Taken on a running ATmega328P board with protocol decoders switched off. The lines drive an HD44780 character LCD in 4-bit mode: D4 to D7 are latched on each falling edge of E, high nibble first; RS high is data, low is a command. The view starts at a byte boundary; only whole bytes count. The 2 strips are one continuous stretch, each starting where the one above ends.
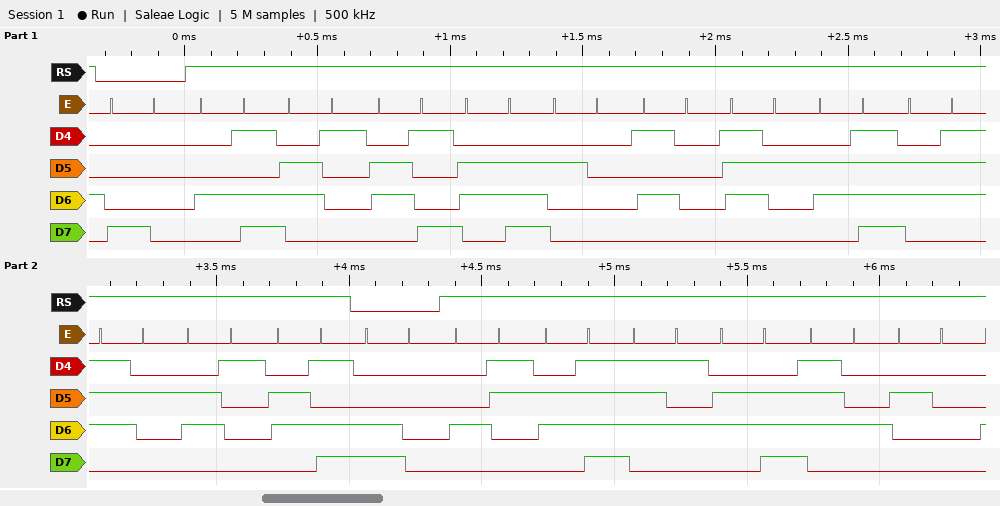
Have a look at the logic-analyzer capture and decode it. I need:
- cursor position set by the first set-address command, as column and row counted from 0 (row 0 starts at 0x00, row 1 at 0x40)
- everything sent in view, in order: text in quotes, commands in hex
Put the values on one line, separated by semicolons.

column 0, row 0; 0x80 "Main Program" 0xC0 "Count "
